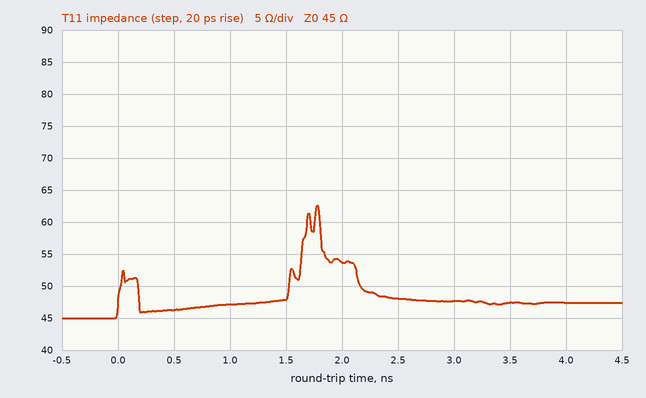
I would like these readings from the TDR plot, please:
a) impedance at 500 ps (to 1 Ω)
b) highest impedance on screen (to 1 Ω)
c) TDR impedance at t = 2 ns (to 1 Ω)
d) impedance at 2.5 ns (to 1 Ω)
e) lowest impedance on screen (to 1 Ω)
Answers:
46 Ω
63 Ω
54 Ω
48 Ω
45 Ω
